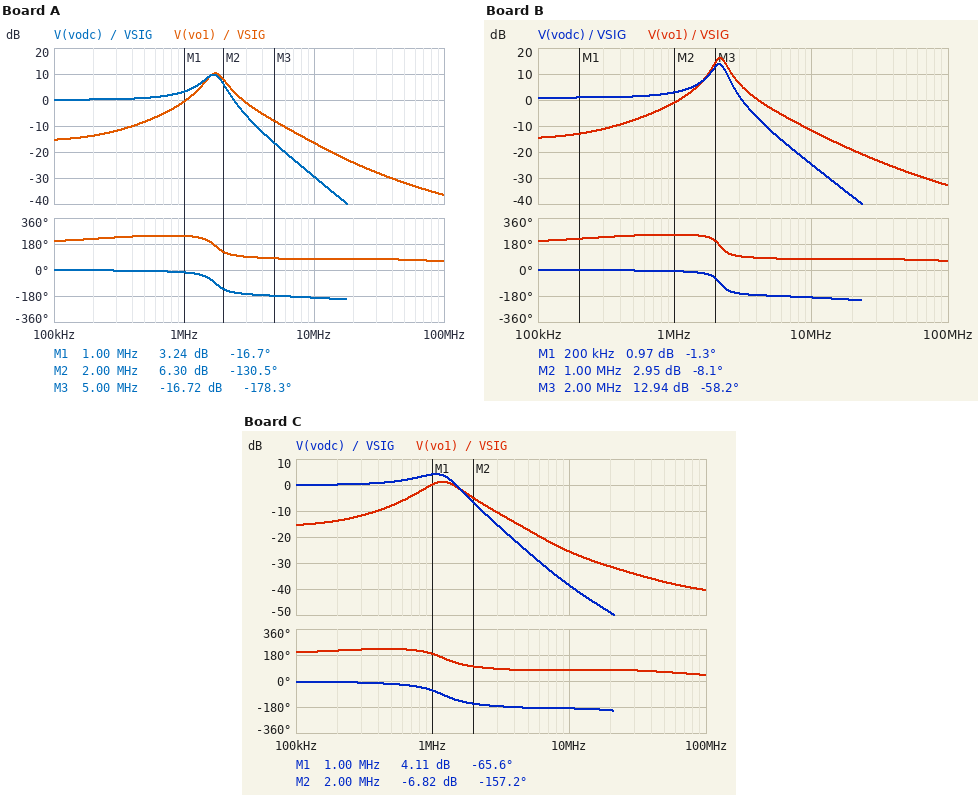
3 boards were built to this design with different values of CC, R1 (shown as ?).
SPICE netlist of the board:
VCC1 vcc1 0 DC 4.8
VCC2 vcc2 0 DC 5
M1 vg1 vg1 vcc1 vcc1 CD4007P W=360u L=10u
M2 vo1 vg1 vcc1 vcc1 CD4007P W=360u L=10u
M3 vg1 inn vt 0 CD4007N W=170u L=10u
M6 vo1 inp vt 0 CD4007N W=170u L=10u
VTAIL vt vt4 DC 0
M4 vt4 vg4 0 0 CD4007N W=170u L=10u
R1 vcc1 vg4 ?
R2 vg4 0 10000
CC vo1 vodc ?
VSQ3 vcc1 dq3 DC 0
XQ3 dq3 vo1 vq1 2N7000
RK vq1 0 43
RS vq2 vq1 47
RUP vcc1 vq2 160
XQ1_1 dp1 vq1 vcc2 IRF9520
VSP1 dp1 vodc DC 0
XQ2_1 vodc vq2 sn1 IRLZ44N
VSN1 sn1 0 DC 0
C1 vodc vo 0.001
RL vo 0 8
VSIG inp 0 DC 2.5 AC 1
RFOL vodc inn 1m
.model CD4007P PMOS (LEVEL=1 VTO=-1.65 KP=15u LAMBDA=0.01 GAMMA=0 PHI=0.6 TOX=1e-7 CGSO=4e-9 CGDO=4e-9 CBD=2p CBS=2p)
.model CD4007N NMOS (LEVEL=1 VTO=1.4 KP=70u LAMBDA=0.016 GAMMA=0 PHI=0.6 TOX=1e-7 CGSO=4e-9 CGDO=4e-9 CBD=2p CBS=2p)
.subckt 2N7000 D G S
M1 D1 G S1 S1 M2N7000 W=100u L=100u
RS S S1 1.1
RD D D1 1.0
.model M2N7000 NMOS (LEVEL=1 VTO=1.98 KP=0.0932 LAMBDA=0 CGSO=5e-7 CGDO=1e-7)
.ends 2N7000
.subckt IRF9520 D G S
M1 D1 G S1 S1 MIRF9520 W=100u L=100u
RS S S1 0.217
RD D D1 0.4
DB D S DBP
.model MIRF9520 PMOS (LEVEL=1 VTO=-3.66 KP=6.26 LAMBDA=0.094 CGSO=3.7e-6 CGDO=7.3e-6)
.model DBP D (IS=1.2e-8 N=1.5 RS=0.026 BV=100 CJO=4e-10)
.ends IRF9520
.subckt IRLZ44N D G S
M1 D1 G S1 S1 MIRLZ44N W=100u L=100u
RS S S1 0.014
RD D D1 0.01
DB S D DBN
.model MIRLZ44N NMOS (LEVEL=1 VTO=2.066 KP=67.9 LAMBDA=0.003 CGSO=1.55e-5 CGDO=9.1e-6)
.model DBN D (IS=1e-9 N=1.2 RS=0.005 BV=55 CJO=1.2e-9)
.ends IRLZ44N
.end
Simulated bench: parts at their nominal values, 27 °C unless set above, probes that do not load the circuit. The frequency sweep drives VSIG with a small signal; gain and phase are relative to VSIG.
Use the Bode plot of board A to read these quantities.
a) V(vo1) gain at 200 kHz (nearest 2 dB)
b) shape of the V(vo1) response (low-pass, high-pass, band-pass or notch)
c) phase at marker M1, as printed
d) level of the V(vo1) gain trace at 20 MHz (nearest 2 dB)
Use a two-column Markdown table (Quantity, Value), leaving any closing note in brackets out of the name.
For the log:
| Quantity | Value |
|---|---|
| V(vo1) gain at 200 kHz | -14 dB |
| shape of the V(vo1) response | band-pass |
| phase at marker M1, as printed | -16.7 deg |
| level of the V(vo1) gain trace at 20 MHz | -24 dB |
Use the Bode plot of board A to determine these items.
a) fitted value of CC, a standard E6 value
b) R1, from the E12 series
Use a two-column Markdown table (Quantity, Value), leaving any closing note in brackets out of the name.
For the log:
| Quantity | Value |
|---|---|
| fitted value of CC, a standard E6 value | 22 pF |
| R1, from the E12 series | 8.2 kΩ |
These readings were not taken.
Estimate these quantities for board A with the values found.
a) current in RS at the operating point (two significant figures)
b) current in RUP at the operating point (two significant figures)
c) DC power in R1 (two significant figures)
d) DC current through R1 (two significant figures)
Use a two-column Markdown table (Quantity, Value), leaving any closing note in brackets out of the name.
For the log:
| Quantity | Value |
|---|---|
| current in RS at the operating point | 17 mA |
| current in RUP at the operating point | 17 mA |
| DC power in R1 | 570 µW |
| DC current through R1 | 260 µA |
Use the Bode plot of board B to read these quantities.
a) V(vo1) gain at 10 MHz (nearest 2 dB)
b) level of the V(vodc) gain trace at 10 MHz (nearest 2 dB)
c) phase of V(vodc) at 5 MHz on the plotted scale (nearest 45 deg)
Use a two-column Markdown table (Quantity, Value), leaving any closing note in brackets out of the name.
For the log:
| Quantity | Value |
|---|---|
| V(vo1) gain at 10 MHz | -12 dB |
| level of the V(vodc) gain trace at 10 MHz | -24 dB |
| phase of V(vodc) at 5 MHz on the plotted scale | -180 deg |
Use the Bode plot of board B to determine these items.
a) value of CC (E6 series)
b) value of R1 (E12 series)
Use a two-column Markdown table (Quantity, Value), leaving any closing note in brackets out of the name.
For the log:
| Quantity | Value |
|---|---|
| value of CC | 3.3 pF |
| value of R1 | 2.7 kΩ |
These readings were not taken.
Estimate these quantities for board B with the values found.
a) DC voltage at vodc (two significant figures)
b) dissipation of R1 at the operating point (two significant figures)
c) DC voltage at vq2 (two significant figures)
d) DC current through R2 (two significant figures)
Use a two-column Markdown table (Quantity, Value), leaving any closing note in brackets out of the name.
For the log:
| Quantity | Value |
|---|---|
| DC voltage at vodc | 2.5 V |
| dissipation of R1 at the operating point | 390 µW |
| DC voltage at vq2 | 2.1 V |
| DC current through R2 | 380 µA |
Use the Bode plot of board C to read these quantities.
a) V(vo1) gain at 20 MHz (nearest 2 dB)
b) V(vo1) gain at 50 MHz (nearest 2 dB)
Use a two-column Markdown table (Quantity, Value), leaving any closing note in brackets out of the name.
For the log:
| Quantity | Value |
|---|---|
| V(vo1) gain at 20 MHz | -32 dB |
| V(vo1) gain at 50 MHz | -38 dB |
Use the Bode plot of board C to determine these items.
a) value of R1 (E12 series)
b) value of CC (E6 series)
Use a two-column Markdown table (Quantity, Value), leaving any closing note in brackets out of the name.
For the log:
| Quantity | Value |
|---|---|
| value of R1 | 15 kΩ |
| value of CC | 33 pF |
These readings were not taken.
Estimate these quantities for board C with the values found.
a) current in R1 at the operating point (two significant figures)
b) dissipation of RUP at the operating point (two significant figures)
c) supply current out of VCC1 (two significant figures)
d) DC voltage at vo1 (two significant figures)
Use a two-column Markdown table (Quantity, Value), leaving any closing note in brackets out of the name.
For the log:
| Quantity | Value |
|---|---|
| current in R1 at the operating point | 190 µA |
| dissipation of RUP at the operating point | 46 mW |
| supply current out of VCC1 | 30 mA |
| DC voltage at vo1 | 3.8 V |
